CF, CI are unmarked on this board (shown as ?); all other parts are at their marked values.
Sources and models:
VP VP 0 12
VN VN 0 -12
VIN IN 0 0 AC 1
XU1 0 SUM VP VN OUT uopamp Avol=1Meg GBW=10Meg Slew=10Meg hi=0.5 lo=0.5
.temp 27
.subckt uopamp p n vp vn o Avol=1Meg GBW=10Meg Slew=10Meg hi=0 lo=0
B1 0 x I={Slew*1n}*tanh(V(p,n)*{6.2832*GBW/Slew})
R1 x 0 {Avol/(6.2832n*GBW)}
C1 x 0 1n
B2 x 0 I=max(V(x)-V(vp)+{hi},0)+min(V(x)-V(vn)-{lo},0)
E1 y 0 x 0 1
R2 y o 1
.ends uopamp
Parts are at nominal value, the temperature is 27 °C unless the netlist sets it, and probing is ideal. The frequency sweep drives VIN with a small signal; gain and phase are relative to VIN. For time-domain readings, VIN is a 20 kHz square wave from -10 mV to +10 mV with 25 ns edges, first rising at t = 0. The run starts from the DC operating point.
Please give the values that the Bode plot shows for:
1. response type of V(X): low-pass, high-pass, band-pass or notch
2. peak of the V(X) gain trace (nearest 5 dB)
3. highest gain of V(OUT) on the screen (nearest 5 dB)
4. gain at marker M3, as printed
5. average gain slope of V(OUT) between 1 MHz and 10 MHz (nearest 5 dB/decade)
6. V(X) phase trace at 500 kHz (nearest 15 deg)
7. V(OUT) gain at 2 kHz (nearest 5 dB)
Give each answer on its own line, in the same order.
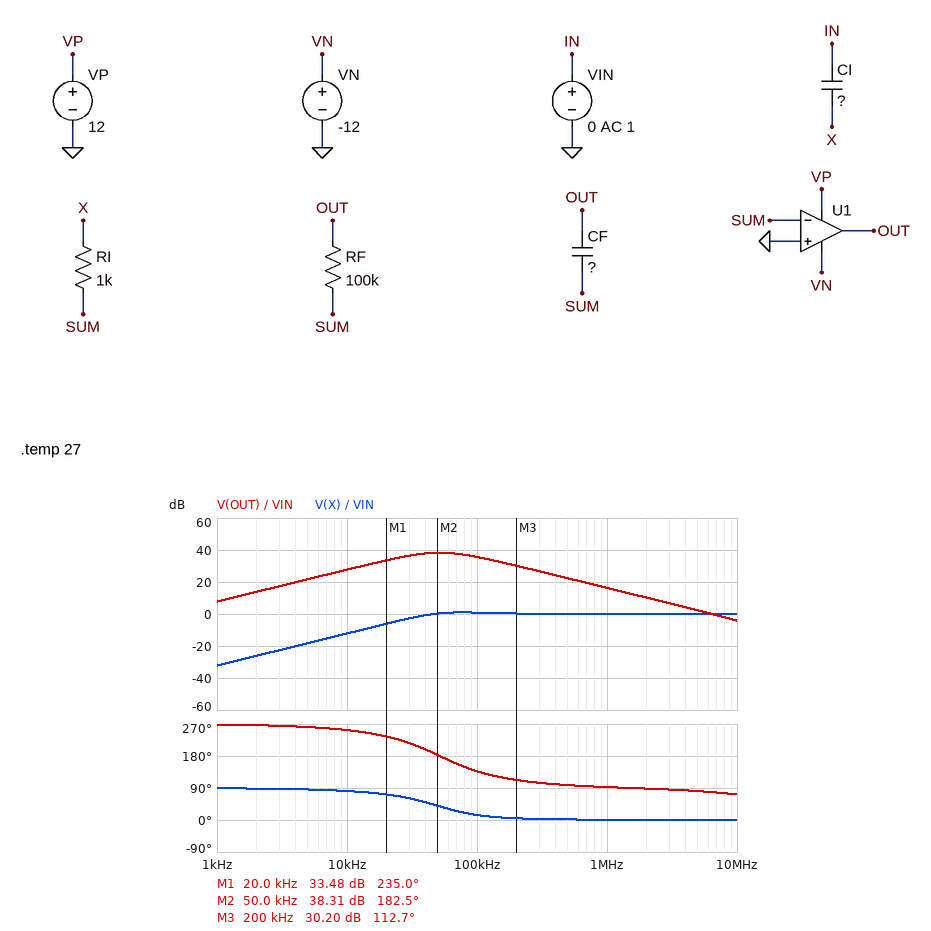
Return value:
high-pass
0 dB
40 dB
30.20 dB
-20 dB/decade
0 deg
15 dB
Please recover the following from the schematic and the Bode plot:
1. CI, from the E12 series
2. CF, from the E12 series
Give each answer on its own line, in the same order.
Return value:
3.9 nF
8.2 pF
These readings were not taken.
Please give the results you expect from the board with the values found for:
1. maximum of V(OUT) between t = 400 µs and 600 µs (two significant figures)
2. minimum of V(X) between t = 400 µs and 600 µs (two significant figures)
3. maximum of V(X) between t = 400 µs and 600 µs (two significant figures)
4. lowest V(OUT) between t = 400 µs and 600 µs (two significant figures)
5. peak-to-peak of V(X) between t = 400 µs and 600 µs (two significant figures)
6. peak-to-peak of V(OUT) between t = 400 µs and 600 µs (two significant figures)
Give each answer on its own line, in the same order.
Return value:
1.1 V
-20 mV
20 mV
-1.1 V
40 mV
2.2 V
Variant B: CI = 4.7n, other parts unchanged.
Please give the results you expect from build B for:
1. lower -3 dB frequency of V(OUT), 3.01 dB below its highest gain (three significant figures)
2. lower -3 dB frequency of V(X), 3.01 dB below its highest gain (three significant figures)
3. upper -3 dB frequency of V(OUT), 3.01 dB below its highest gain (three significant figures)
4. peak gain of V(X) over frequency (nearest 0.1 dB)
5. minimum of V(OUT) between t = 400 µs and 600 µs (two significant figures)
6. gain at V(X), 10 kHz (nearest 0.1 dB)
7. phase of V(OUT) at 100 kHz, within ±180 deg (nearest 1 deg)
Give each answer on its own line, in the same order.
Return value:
22.3 kHz
28.8 kHz
99.6 kHz
0.9 dB
-1.2 V
-10.6 dB
135 deg
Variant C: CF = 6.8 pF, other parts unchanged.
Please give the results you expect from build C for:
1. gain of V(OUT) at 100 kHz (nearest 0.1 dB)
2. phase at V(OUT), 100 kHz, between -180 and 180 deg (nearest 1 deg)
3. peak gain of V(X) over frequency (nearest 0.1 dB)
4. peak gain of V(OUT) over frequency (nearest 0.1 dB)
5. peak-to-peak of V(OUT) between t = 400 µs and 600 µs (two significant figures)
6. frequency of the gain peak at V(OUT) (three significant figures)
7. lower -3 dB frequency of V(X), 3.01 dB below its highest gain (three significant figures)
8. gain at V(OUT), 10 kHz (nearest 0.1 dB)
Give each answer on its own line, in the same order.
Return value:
36.1 dB
139 deg
1.1 dB
38.6 dB
2.3 V
53.3 kHz
33.8 kHz
27.7 dB
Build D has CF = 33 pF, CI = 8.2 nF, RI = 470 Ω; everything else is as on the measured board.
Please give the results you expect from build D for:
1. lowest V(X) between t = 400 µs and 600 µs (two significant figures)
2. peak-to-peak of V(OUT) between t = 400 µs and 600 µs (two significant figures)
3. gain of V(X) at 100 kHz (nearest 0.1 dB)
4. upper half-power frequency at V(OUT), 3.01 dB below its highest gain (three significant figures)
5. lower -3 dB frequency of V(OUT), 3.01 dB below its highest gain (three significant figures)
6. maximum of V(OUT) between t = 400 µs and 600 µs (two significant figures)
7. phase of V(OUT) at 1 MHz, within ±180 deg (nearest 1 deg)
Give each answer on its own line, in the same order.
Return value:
-21 mV
3.1 V
0.2 dB
60.4 kHz
16.2 kHz
1.5 V
90 deg
